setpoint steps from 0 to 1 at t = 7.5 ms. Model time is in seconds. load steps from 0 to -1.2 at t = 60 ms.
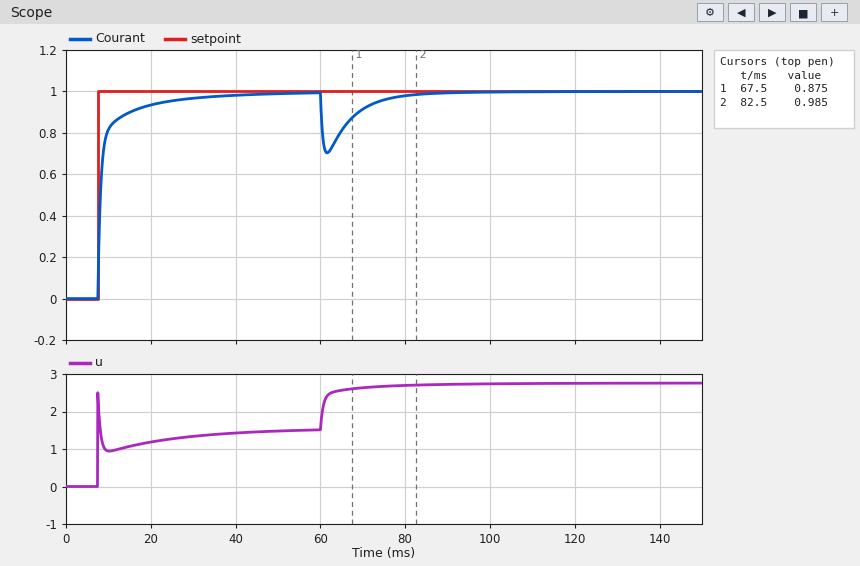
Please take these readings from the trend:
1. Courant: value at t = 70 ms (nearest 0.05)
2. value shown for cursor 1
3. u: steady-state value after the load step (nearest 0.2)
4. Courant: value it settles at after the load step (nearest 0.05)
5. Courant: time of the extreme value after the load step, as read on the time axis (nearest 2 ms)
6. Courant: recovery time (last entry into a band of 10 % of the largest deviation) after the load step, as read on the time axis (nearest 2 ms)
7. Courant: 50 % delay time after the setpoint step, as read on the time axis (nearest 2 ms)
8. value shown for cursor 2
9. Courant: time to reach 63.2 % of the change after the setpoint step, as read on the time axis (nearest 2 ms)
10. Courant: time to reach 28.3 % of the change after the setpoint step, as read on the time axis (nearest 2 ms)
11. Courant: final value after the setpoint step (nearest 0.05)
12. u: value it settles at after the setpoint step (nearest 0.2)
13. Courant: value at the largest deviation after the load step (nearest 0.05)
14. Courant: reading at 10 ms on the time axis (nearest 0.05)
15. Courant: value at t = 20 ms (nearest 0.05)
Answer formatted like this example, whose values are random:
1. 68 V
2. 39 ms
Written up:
1. 0.90
2. 0.875
3. 2.8
4. 1.00
5. 62 ms
6. 78 ms
7. 8 ms
8. 0.985
9. 8 ms
10. 8 ms
11. 1.00
12. 1.6
13. 0.70
14. 0.80
15. 0.95
